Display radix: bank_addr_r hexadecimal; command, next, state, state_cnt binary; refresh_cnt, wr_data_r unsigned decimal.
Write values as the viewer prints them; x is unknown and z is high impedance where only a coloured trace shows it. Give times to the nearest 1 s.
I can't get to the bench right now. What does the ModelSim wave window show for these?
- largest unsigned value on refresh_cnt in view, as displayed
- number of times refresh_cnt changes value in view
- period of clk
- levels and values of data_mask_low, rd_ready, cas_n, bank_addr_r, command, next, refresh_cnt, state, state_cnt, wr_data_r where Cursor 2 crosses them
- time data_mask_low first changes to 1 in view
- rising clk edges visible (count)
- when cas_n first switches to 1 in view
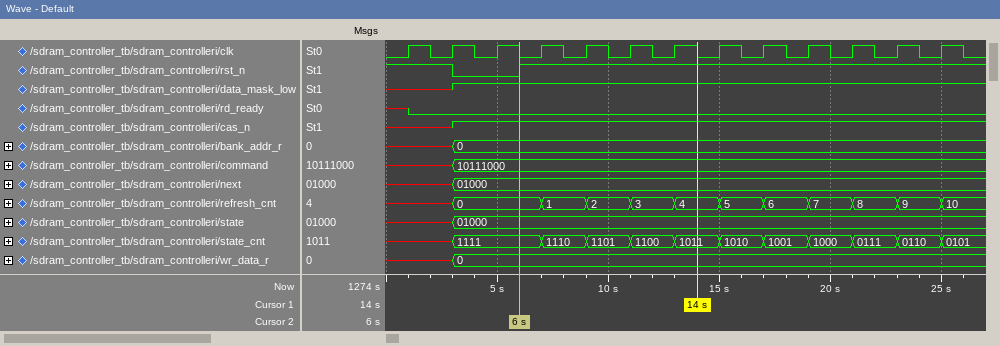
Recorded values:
10
11
2 s
data_mask_low=1, rd_ready=0, cas_n=1, bank_addr_r=0, command=10111000, next=01000, refresh_cnt=0, state=01000, state_cnt=1111, wr_data_r=0
3 s
13
3 s
